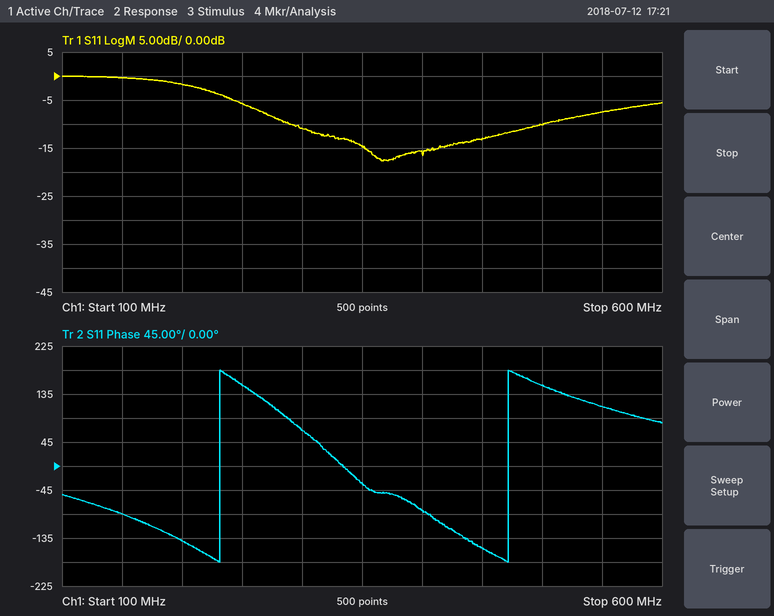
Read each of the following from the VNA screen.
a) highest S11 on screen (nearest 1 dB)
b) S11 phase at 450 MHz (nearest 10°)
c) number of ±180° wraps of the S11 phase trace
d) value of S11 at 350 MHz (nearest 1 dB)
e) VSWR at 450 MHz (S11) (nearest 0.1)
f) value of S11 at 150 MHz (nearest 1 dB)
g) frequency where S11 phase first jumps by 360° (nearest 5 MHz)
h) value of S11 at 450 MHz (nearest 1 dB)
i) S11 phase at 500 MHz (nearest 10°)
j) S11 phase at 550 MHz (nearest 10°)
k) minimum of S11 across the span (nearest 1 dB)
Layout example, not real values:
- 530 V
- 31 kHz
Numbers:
- 0 dB
- -150°
- 2
- -15 dB
- 1.6
- 0 dB
- 230 MHz
- -13 dB
- 150°
- 110°
- -18 dB
